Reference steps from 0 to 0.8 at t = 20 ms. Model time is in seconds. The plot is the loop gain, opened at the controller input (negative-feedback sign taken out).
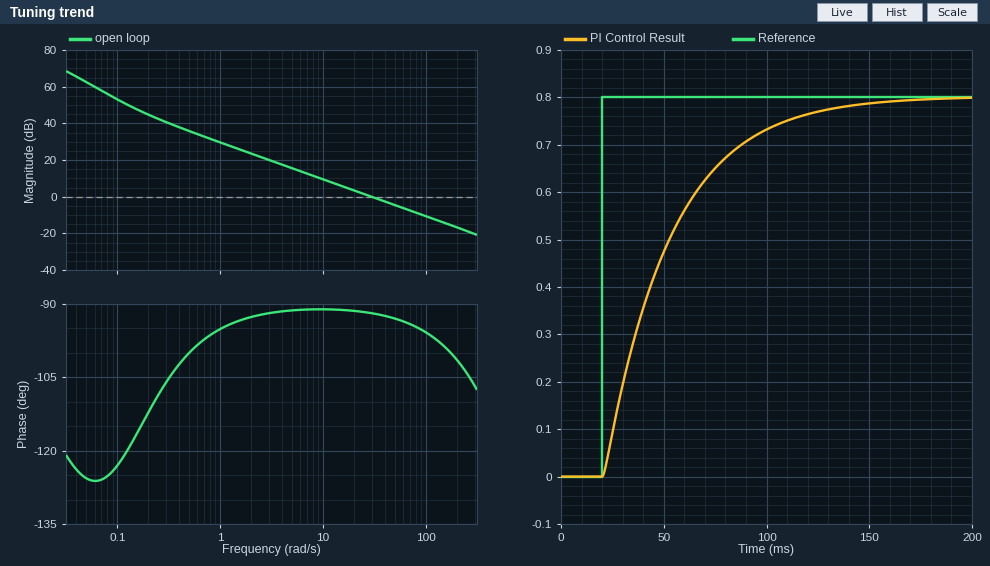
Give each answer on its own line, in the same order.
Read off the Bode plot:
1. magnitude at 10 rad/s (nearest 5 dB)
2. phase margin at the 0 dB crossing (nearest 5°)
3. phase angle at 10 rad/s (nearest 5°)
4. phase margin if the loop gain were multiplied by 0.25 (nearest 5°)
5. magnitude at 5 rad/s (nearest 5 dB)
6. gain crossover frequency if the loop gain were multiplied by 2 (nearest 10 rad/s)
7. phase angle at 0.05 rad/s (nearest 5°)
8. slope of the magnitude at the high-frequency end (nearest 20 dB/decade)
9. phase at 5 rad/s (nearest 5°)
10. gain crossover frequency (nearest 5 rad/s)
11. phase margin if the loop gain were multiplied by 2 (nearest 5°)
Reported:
10 dB
90°
-90°
90°
15 dB
60 rad/s
-125°
-20 dB/decade
-90°
30 rad/s
85°
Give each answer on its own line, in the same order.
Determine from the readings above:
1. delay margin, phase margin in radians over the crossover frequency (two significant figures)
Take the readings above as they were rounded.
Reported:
0.052 s
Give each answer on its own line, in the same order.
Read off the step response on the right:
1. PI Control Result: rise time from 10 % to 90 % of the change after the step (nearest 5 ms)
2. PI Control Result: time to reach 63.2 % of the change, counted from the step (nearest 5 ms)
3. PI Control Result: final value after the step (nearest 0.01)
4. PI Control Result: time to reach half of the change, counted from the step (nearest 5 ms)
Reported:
70 ms
35 ms
0.80
25 ms
